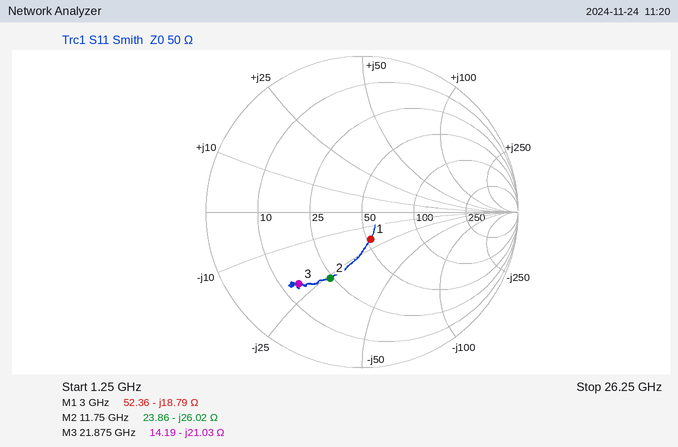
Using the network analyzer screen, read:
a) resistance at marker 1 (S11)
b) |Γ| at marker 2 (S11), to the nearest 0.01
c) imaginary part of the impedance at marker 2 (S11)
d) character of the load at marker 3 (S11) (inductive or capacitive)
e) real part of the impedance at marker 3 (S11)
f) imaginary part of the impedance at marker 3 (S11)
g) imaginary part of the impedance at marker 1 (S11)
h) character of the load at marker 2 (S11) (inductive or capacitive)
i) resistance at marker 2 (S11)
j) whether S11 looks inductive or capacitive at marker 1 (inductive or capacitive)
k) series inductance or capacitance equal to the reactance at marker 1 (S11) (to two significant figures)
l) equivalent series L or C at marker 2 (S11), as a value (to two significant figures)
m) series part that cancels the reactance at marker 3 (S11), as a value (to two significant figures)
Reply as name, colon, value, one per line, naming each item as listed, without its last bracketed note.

resistance at marker 1: 52.36 Ω
|Γ| at marker 2 (S11), to the nearest 0.01: 0.47
imaginary part of the impedance at marker 2: -26.02 Ω
character of the load at marker 3 (S11): capacitive
real part of the impedance at marker 3: 14.19 Ω
imaginary part of the impedance at marker 3: -21.03 Ω
imaginary part of the impedance at marker 1: -18.79 Ω
character of the load at marker 2 (S11): capacitive
resistance at marker 2: 23.86 Ω
whether S11 looks inductive or capacitive at marker 1: capacitive
series inductance or capacitance equal to the reactance at marker 1 (S11): 2.8 pF
equivalent series L or C at marker 2 (S11), as a value: 520 fF
series part that cancels the reactance at marker 3 (S11), as a value: 150 pH
